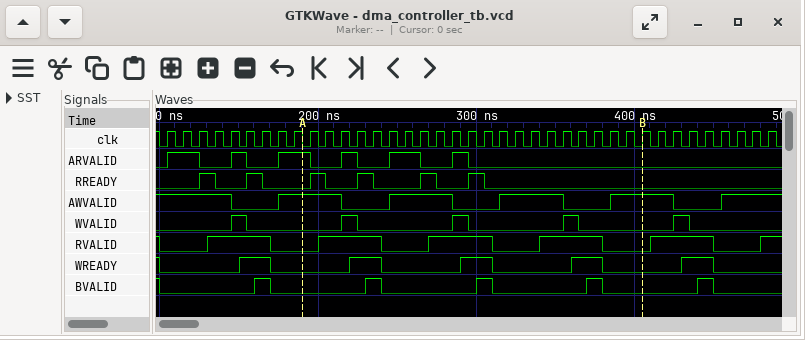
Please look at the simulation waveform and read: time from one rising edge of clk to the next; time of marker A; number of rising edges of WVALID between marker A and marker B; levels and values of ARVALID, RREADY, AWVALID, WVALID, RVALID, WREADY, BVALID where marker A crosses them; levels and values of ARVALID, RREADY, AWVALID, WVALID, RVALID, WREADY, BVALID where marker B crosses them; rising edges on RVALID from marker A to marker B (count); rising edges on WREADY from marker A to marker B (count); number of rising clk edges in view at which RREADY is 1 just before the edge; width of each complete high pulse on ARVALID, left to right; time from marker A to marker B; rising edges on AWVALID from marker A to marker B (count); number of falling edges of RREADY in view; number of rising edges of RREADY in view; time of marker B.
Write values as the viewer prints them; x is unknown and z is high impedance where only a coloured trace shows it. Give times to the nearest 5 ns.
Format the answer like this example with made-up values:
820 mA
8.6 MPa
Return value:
10 ns
190 ns
3
ARVALID=1, RREADY=0, AWVALID=1, WVALID=0, RVALID=0, WREADY=0, BVALID=0
ARVALID=0, RREADY=0, AWVALID=1, WVALID=0, RVALID=0, WREADY=0, BVALID=0
3
3
6
20 ns, 10 ns, 20 ns, 10 ns, 20 ns, 10 ns
215 ns
3
6
6
405 ns
